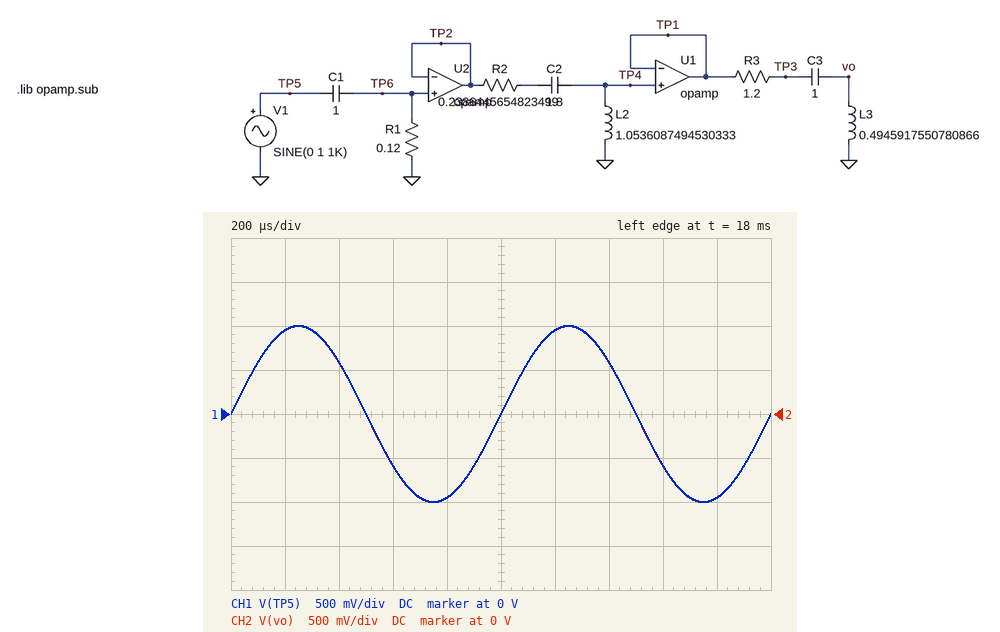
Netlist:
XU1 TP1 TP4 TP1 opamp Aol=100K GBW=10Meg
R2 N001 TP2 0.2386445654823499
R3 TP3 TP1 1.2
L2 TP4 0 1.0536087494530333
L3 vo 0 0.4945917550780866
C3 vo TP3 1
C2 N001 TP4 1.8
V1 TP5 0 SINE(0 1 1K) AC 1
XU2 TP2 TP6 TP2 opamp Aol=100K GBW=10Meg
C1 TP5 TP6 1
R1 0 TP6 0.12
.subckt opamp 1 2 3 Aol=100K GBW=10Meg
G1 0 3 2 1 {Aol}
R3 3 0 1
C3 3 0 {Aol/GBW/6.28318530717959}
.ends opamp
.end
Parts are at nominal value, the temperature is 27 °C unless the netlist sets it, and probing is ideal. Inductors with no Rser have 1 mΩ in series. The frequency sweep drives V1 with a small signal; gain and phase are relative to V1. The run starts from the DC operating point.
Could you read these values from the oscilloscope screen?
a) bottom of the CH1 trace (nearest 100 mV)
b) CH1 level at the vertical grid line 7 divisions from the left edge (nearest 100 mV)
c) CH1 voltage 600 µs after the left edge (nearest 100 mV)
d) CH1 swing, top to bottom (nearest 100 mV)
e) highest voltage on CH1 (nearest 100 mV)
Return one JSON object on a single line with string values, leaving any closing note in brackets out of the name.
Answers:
{"bottom of the CH1 trace": "-1.0 V", "CH1 level at the vertical grid line 7 divisions from the left edge": "600 mV", "CH1 voltage 600 µs after the left edge": "-600 mV", "CH1 swing, top to bottom": "2.0 V", "highest voltage on CH1": "1.0 V"}
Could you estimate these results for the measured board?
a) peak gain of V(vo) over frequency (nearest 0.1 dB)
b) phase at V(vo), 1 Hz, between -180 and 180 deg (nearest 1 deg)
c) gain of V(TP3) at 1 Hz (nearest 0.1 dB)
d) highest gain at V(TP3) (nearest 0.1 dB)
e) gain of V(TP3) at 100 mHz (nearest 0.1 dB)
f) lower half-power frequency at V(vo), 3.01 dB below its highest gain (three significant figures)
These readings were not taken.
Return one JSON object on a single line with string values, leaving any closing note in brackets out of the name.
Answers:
{"peak gain of V(vo) over frequency": "0 dB", "phase at V(vo), 1 Hz, between -180 and 180 deg": "77 deg", "gain of V(TP3) at 1 Hz": "-5.0 dB", "highest gain at V(TP3)": "0 dB", "gain of V(TP3) at 100 mHz": "-19.1 dB", "lower half-power frequency at V(vo), 3.01 dB below its highest gain": "1.34 Hz"}
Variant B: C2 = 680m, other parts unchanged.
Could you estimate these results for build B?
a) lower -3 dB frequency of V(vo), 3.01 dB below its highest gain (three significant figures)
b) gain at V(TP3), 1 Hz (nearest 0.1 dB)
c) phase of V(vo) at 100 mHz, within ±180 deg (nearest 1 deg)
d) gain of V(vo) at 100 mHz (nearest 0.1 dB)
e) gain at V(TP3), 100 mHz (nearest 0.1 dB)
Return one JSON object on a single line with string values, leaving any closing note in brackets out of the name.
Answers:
{"lower -3 dB frequency of V(vo), 3.01 dB below its highest gain": "1.31 Hz", "gain at V(TP3), 1 Hz": "-4.8 dB", "phase of V(vo) at 100 mHz, within ±180 deg": "34 deg", "gain of V(vo) at 100 mHz": "-45.7 dB", "gain at V(TP3), 100 mHz": "-33.4 dB"}
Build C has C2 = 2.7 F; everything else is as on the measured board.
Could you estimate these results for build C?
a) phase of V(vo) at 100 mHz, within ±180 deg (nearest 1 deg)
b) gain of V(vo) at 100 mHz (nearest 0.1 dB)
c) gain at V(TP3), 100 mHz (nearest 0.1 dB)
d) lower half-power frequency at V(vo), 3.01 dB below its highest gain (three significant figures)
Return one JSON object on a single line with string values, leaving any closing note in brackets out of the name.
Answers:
{"phase of V(vo) at 100 mHz, within ±180 deg": "-65 deg", "gain of V(vo) at 100 mHz": "-29.1 dB", "gain at V(TP3), 100 mHz": "-16.8 dB", "lower half-power frequency at V(vo), 3.01 dB below its highest gain": "1.35 Hz"}
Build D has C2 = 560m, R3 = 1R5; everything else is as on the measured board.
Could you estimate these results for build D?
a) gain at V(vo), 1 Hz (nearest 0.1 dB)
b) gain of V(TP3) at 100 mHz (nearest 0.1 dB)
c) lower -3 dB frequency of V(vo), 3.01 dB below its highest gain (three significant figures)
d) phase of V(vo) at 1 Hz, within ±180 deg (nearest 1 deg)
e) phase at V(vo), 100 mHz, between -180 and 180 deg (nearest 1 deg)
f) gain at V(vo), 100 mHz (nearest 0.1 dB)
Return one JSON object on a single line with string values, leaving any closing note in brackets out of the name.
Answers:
{"gain at V(vo), 1 Hz": "-4.6 dB", "gain of V(TP3) at 100 mHz": "-36.6 dB", "lower -3 dB frequency of V(vo), 3.01 dB below its highest gain": "1.36 Hz", "phase of V(vo) at 1 Hz, within ±180 deg": "82 deg", "phase at V(vo), 100 mHz, between -180 and 180 deg": "30 deg", "gain at V(vo), 100 mHz": "-48.9 dB"}
